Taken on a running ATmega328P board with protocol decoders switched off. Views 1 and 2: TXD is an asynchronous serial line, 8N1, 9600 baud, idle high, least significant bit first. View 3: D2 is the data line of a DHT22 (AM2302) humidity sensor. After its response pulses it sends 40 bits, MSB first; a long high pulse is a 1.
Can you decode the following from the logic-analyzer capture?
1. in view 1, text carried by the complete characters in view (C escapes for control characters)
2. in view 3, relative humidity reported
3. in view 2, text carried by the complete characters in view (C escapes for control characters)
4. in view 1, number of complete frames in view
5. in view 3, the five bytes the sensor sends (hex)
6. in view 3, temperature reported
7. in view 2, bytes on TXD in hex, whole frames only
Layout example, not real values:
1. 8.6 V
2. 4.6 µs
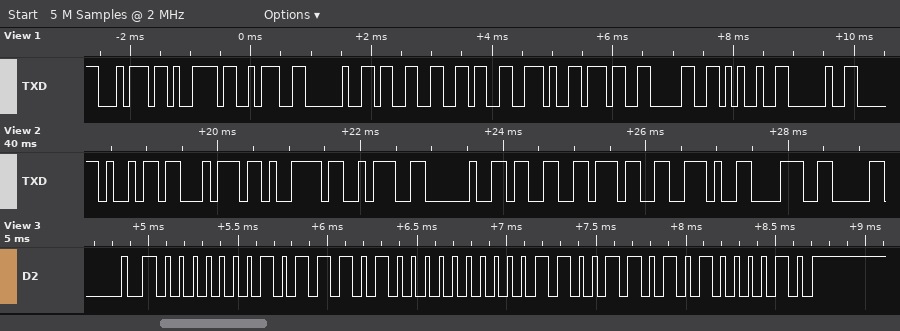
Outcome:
1. "ty: 36.70% "
2. 37.2 %
3. "ity: 37.8"
4. 11
5. 01 74 00 CD 42
6. 20.5 °C
7. 0x69 0x74 0x79 0x3A 0x20 0x33 0x37 0x2E 0x38
